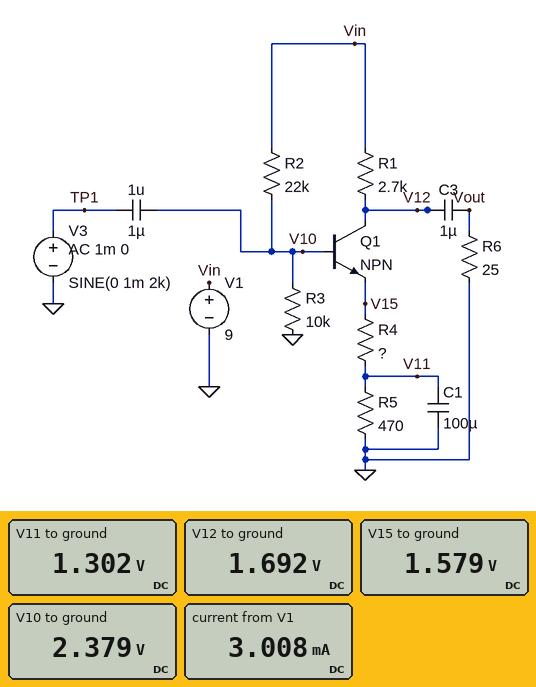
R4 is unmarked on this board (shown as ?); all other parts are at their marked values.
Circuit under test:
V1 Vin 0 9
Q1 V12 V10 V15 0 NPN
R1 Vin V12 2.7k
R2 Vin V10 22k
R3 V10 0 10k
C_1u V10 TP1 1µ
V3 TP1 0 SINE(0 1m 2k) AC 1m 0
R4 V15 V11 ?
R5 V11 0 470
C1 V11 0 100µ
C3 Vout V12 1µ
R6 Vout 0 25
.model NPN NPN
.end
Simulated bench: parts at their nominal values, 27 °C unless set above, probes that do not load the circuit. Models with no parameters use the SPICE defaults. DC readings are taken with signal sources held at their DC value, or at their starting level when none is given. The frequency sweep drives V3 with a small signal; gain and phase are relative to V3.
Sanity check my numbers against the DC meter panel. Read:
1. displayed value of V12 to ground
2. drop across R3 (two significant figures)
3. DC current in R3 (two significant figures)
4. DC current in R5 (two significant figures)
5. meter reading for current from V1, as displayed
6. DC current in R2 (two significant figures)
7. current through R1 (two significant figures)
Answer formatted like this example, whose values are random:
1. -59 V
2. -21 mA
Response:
1. 1.692 V
2. 2.4 V
3. 240 µA
4. 2.8 mA
5. 3.008 mA
6. 300 µA
7. 2.7 mA
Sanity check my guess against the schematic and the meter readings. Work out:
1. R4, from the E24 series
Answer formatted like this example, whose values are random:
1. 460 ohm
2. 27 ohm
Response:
1. 100 Ω
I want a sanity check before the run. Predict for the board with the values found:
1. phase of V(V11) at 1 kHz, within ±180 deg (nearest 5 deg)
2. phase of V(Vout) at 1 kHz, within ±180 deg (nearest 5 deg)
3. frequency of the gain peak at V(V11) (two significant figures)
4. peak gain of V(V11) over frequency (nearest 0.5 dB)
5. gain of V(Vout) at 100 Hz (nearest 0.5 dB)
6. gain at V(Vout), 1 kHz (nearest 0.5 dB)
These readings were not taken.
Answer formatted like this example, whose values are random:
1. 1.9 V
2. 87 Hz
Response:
1. -65 deg
2. -140 deg
3. 550 Hz
4. -31.5 dB
5. -45.0 dB
6. -14.0 dB
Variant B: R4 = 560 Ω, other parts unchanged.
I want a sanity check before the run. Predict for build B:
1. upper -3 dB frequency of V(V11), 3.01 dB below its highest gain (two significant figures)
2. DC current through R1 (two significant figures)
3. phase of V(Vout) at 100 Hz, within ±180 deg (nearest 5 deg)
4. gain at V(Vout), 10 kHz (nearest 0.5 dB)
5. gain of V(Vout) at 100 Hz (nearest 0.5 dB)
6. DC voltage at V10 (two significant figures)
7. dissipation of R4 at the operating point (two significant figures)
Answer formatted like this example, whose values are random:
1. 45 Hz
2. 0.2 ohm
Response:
1. 36 Hz
2. 1.8 mA
3. -135 deg
4. -27.5 dB
5. -29.0 dB
6. 2.7 V
7. 1.9 mW
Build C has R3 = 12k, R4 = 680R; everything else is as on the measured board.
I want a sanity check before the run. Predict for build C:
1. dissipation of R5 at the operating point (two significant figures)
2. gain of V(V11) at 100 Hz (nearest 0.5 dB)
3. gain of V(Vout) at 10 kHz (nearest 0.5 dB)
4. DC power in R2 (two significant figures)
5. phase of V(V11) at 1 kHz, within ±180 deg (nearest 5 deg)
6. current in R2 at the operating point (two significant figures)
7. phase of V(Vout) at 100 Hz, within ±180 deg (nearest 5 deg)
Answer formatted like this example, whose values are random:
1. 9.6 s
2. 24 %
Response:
1. 1.8 mW
2. -33.0 dB
3. -29.0 dB
4. 1.6 mW
5. -90 deg
6. 270 µA
7. -135 deg
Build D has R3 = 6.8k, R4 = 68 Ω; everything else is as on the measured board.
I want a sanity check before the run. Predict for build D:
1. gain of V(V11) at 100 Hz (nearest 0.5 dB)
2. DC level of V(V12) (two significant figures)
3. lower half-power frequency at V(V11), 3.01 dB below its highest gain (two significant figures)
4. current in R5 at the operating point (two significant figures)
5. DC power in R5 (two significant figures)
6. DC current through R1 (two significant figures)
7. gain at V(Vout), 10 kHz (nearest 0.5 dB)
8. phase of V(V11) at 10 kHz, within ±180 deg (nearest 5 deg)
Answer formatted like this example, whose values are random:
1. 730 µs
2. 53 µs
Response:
1. -15.5 dB
2. 3.0 V
3. 9.4 Hz
4. 2.3 mA
5. 2.4 mW
6. 2.2 mA
7. -10.0 dB
8. -90 deg
